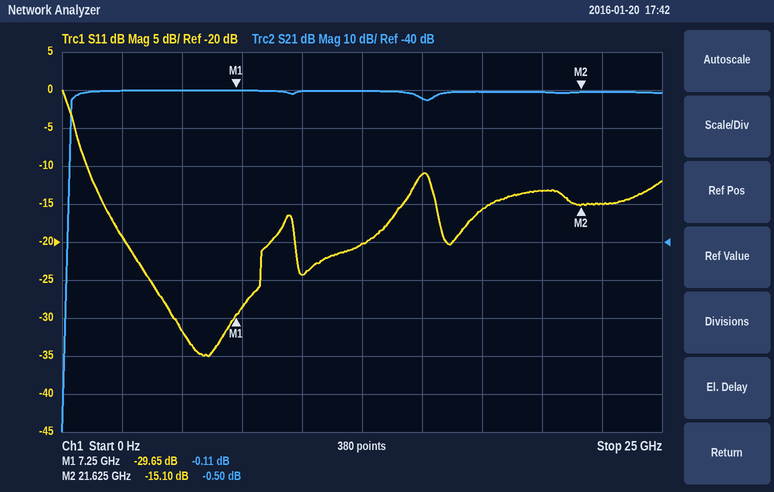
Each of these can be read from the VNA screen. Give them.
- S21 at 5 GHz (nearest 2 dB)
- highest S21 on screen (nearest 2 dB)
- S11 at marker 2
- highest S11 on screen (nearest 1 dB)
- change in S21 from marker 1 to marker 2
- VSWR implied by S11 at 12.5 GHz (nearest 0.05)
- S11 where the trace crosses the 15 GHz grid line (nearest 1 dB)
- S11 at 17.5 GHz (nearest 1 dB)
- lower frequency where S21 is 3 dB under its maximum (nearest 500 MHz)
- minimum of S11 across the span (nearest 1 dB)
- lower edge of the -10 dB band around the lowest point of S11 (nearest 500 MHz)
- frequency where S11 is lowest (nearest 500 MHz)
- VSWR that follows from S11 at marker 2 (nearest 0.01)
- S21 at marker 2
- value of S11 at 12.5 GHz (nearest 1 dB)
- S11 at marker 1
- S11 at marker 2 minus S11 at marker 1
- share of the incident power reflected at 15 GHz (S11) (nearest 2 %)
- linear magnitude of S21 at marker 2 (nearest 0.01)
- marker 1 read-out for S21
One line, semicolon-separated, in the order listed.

0 dB; 0 dB; -15.10 dB; 0 dB; -0.39 dB; 1.20; -11 dB; -16 dB; 500 MHz; -35 dB; 1.0 GHz; 6.0 GHz; 1.43; -0.50 dB; -20 dB; -29.65 dB; 14.55 dB; 8 %; 0.94; -0.11 dB
